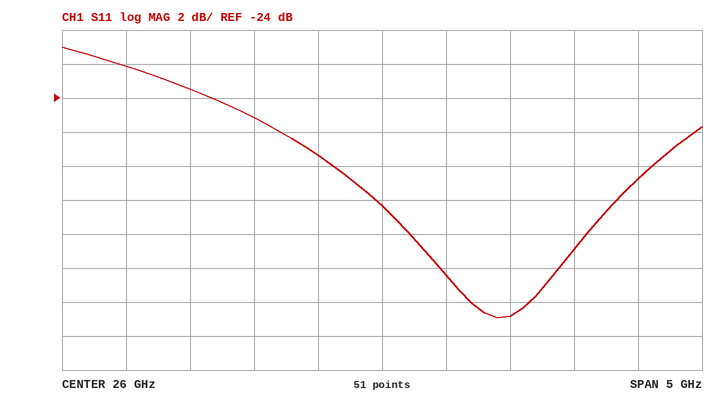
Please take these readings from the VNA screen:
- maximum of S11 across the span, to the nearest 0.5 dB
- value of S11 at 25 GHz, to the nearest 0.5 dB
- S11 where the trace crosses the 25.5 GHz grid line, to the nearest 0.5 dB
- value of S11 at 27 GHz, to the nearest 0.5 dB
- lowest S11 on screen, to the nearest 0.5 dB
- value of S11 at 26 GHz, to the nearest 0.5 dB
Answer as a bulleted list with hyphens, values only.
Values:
- -21.0 dB
- -25.0 dB
- -27.5 dB
- -37.0 dB
- -37.0 dB
- -30.5 dB
